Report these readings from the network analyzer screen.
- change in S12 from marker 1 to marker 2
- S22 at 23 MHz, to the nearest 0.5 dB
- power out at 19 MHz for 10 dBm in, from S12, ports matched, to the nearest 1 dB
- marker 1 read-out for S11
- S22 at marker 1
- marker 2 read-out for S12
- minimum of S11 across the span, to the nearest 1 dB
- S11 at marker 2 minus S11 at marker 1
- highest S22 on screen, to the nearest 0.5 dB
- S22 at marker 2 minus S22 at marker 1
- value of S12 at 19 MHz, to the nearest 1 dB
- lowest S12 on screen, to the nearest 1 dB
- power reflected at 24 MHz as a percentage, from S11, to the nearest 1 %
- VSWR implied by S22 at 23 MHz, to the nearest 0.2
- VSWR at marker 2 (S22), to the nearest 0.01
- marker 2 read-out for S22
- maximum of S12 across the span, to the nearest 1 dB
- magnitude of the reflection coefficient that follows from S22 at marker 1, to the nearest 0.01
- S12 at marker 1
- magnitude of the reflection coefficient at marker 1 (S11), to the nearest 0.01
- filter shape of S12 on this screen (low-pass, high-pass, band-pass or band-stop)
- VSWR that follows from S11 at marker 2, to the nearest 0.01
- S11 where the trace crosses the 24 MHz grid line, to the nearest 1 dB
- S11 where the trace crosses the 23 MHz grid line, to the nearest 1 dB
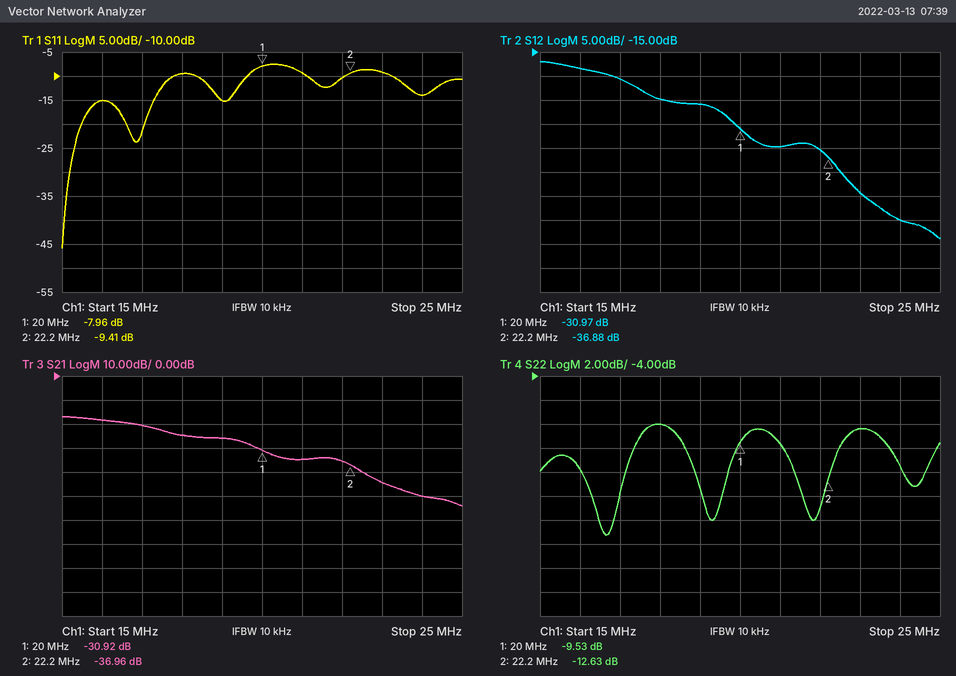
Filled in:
-5.91 dB
-8.5 dB
-16 dBm
-7.96 dB
-9.53 dB
-36.88 dB
-46 dB
-1.45 dB
-8.0 dB
-3.10 dB
-26 dB
-54 dB
4 %
2.2
1.61
-12.63 dB
-17 dB
0.33
-30.97 dB
0.40
low-pass
2.02
-14 dB
-9 dB
